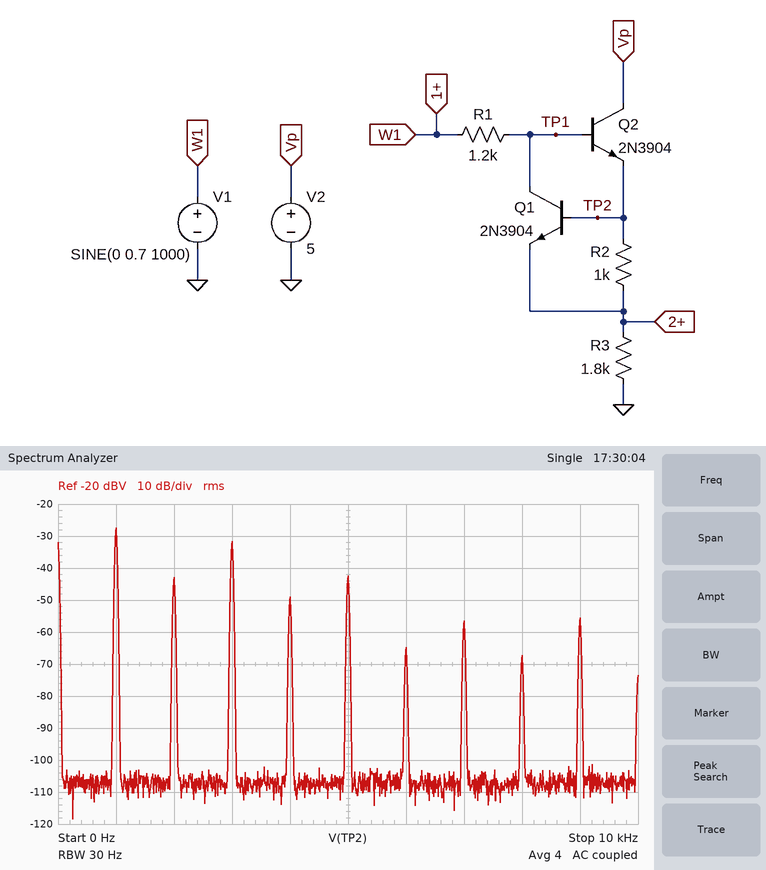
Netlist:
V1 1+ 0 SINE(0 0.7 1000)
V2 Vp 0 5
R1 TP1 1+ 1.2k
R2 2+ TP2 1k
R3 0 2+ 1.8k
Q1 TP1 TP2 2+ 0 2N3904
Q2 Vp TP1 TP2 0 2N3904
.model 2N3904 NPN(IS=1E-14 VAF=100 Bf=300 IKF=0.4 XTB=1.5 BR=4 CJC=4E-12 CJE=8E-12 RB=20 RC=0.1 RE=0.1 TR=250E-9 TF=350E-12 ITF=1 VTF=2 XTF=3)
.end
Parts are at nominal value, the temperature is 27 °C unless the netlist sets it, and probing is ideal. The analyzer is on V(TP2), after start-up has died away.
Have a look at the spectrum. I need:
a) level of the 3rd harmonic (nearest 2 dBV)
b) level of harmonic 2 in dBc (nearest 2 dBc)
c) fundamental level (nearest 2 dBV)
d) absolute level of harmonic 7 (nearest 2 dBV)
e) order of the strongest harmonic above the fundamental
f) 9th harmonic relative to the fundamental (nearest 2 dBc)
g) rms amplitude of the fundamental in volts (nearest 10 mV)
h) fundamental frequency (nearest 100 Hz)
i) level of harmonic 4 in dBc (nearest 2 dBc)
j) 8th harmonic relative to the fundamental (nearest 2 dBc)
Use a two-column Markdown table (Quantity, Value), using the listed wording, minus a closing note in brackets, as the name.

| Quantity | Value |
|---|---|
| level of the 3rd harmonic | -32 dBV |
| level of harmonic 2 in dBc | -16 dBc |
| fundamental level | -28 dBV |
| absolute level of harmonic 7 | -56 dBV |
| order of the strongest harmonic above the fundamental | 3 |
| 9th harmonic relative to the fundamental | -28 dBc |
| rms amplitude of the fundamental in volts | 40 mV |
| fundamental frequency | 1.0 kHz |
| level of harmonic 4 in dBc | -22 dBc |
| 8th harmonic relative to the fundamental | -40 dBc |
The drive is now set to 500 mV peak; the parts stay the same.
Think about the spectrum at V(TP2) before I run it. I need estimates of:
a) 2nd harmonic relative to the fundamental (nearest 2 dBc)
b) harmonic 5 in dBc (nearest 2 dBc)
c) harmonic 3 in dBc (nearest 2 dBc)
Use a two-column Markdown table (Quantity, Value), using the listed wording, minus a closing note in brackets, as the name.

| Quantity | Value |
|---|---|
| 2nd harmonic relative to the fundamental | -20 dBc |
| harmonic 5 in dBc | -6 dBc |
| harmonic 3 in dBc | -2 dBc |
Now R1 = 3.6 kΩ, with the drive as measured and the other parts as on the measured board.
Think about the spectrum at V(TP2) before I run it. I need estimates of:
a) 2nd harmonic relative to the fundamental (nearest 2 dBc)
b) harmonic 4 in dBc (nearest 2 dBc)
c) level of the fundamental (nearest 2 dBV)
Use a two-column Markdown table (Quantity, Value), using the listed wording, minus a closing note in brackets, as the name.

| Quantity | Value |
|---|---|
| 2nd harmonic relative to the fundamental | -10 dBc |
| harmonic 4 in dBc | -16 dBc |
| level of the fundamental | -28 dBV |
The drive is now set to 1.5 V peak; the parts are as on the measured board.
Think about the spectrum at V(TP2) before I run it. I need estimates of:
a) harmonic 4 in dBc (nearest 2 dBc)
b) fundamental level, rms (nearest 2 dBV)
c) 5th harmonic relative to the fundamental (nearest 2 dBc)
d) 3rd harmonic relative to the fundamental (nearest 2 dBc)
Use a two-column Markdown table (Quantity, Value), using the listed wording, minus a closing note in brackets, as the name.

| Quantity | Value |
|---|---|
| harmonic 4 in dBc | -56 dBc |
| fundamental level, rms | -8 dBV |
| 5th harmonic relative to the fundamental | -22 dBc |
| 3rd harmonic relative to the fundamental | -12 dBc |
